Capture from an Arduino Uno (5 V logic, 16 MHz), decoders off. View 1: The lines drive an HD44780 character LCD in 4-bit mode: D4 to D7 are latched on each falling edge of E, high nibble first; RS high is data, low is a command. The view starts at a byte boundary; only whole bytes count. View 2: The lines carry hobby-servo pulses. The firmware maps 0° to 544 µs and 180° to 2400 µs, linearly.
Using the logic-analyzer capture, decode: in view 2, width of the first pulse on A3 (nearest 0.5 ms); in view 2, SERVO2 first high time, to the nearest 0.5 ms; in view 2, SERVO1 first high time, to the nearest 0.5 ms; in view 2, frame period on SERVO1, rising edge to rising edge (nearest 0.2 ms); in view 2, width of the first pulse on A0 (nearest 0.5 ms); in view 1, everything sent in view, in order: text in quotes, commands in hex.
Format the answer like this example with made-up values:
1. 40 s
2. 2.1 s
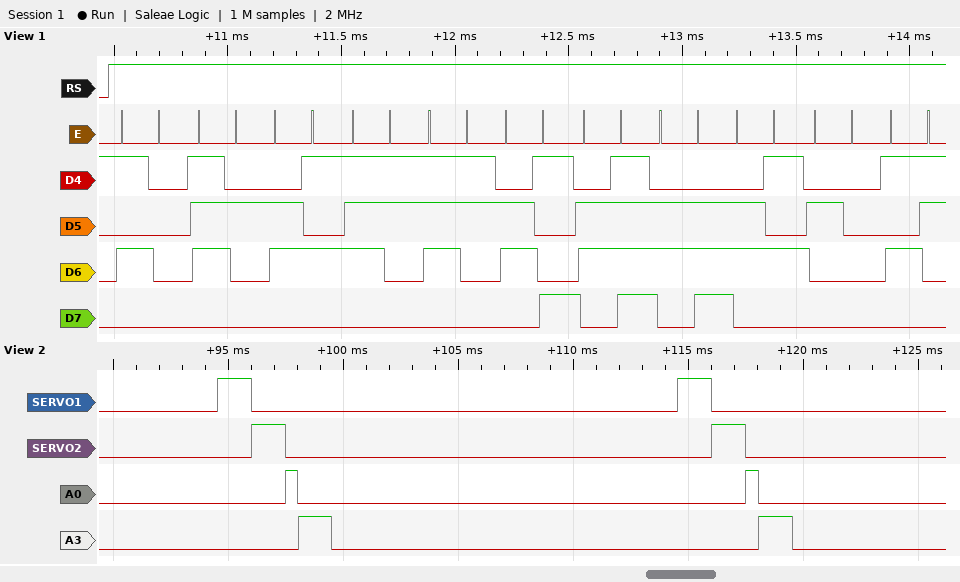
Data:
1. 1.5 ms
2. 1.5 ms
3. 1.5 ms
4. 20.0 ms
5. 0.5 ms
6. "Pressione S"
